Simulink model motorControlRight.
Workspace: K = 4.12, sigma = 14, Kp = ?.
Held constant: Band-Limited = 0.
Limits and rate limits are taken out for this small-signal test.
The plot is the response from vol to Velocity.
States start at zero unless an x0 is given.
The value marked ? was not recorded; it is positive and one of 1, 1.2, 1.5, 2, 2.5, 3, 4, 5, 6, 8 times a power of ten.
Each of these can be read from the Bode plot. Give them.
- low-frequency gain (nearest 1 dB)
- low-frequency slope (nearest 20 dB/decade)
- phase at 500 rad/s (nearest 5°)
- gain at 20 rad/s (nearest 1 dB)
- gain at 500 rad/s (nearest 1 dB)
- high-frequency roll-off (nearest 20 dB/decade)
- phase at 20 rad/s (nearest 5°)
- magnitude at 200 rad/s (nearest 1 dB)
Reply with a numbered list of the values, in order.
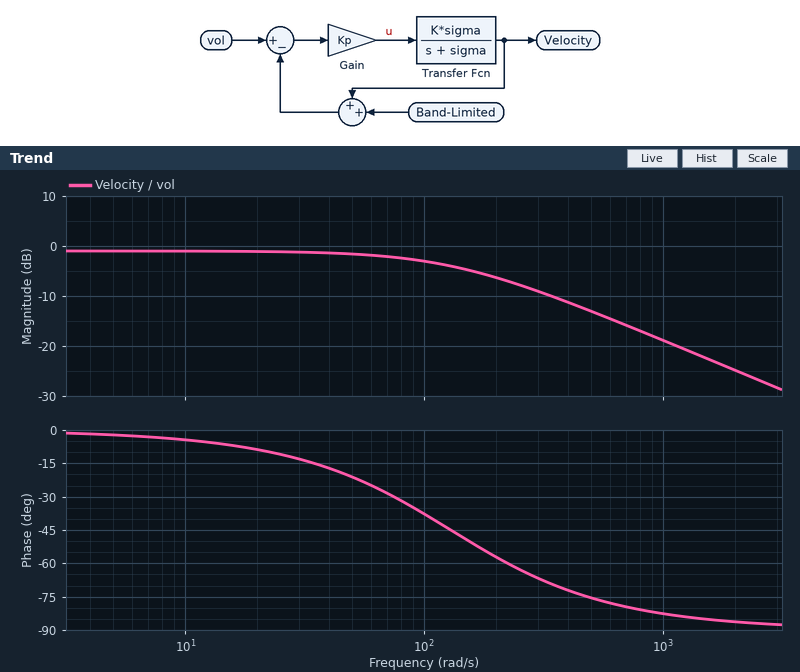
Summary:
1. -1 dB
2. 0 dB/decade
3. -75°
4. -1 dB
5. -13 dB
6. -20 dB/decade
7. -10°
8. -6 dB
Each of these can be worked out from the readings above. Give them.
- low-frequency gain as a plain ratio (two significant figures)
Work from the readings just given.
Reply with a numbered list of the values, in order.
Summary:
1. 0.89
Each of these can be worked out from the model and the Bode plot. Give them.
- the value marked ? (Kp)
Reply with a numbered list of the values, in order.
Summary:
1. 2
